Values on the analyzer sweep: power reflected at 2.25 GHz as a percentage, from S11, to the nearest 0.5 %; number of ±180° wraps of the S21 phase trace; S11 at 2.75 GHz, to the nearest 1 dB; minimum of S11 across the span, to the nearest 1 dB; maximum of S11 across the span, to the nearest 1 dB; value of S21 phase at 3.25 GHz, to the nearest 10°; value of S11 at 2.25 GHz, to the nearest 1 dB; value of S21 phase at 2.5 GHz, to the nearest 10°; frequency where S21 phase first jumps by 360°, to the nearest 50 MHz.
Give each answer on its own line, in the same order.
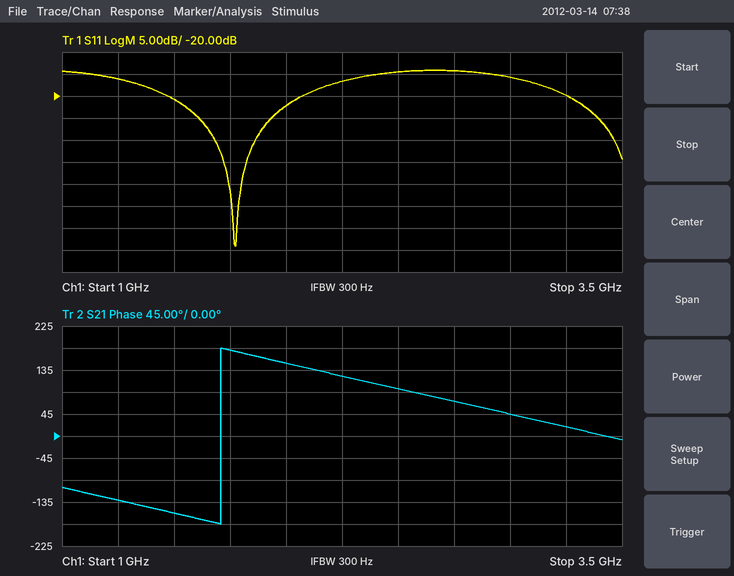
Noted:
2.0 %
1
-14 dB
-54 dB
-14 dB
20°
-17 dB
100°
1.70 GHz
